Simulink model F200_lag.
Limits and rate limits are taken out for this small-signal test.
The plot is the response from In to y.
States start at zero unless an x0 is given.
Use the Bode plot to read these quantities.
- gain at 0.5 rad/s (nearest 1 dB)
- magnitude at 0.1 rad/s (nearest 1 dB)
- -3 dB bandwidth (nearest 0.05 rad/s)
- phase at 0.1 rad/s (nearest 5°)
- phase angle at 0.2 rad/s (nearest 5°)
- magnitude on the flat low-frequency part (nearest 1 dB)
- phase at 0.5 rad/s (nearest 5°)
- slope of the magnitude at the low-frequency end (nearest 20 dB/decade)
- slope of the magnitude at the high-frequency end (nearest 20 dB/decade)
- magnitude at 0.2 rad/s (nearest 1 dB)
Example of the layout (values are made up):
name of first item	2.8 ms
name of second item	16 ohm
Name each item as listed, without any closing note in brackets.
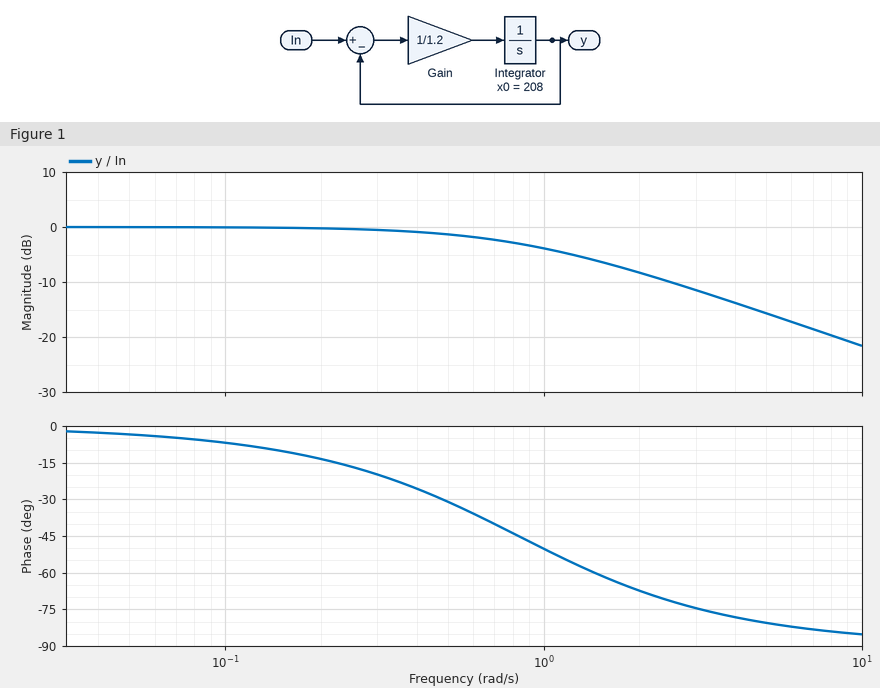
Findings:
gain at 0.5 rad/s	-1 dB
magnitude at 0.1 rad/s	0 dB
-3 dB bandwidth	0.85 rad/s
phase at 0.1 rad/s	-5°
phase angle at 0.2 rad/s	-15°
magnitude on the flat low-frequency part	0 dB
phase at 0.5 rad/s	-30°
slope of the magnitude at the low-frequency end	0 dB/decade
slope of the magnitude at the high-frequency end	-20 dB/decade
magnitude at 0.2 rad/s	0 dB
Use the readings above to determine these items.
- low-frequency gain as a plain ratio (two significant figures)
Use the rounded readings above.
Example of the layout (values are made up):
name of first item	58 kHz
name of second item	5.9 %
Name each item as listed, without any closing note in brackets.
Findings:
low-frequency gain as a plain ratio	1.0
